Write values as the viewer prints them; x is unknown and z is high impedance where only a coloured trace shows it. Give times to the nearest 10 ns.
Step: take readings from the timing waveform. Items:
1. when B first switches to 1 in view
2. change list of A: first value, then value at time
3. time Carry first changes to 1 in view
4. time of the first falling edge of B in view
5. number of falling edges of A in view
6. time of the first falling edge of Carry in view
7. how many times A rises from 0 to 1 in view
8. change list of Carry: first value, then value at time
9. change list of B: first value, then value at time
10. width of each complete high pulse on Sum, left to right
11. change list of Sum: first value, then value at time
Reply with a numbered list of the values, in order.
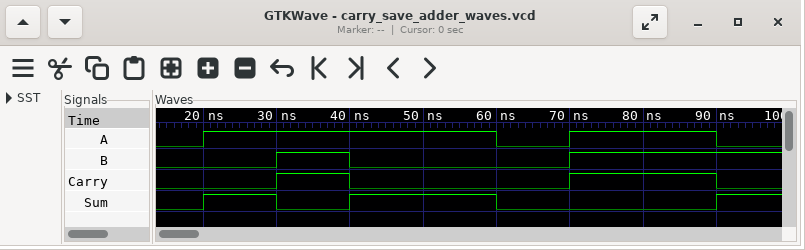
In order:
1. 30 ns
2. 0, 1 at 20 ns, 0 at 60 ns, 1 at 70 ns, 0 at 90 ns
3. 30 ns
4. 40 ns
5. 2
6. 40 ns
7. 2
8. 0, 1 at 30 ns, 0 at 40 ns, 1 at 70 ns, 0 at 90 ns
9. 0, 1 at 30 ns, 0 at 40 ns, 1 at 70 ns
10. 10 ns, 20 ns
11. 0, 1 at 20 ns, 0 at 30 ns, 1 at 40 ns, 0 at 60 ns, 1 at 90 ns
